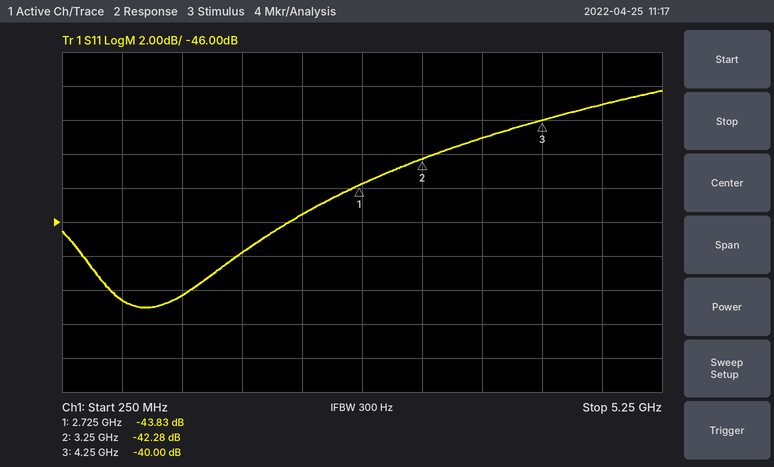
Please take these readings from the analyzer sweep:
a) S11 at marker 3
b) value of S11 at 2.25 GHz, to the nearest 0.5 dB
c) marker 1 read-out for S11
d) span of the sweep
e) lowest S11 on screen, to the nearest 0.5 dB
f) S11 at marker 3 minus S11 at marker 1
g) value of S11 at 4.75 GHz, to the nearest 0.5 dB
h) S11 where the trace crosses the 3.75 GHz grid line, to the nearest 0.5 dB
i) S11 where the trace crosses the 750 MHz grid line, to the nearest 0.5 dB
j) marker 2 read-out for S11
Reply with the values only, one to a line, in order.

-40.00 dB
-45.5 dB
-43.83 dB
5 GHz
-51.0 dB
3.83 dB
-39.0 dB
-41.0 dB
-50.5 dB
-42.28 dB
